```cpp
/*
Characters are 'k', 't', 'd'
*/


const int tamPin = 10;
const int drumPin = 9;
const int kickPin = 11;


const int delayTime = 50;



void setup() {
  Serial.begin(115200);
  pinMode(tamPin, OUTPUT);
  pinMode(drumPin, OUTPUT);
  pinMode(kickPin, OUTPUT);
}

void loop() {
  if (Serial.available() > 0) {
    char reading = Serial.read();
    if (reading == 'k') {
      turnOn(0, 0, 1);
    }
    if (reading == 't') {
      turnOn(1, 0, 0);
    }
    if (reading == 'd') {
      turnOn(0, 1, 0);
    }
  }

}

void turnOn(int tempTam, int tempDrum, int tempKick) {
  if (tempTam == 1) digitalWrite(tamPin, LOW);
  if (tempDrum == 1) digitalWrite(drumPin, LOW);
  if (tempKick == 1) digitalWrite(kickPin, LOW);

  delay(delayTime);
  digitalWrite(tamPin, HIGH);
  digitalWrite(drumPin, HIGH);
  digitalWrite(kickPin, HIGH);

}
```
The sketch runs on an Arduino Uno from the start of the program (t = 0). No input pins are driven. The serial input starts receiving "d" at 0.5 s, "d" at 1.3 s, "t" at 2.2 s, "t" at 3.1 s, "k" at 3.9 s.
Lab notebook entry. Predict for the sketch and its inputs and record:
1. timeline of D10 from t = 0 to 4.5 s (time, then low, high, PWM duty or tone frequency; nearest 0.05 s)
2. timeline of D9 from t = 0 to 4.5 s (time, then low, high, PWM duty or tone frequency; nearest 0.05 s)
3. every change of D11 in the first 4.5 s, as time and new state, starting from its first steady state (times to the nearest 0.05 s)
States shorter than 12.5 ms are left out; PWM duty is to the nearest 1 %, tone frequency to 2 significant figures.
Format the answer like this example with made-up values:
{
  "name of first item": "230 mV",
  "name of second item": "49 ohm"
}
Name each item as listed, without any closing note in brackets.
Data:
{
  "timeline of D10 from t = 0 to 4.5 s": "0 s low; 0.55 s high; 2.2 s low; 2.25 s high; 3.1 s low; 3.15 s high",
  "timeline of D9 from t = 0 to 4.5 s": "0 s low; 0.55 s high; 1.3 s low; 1.35 s high",
  "every change of D11 in the first 4.5 s, as time and new state, starting from its first steady state": "0 s low; 0.55 s high; 3.9 s low; 3.95 s high"
}
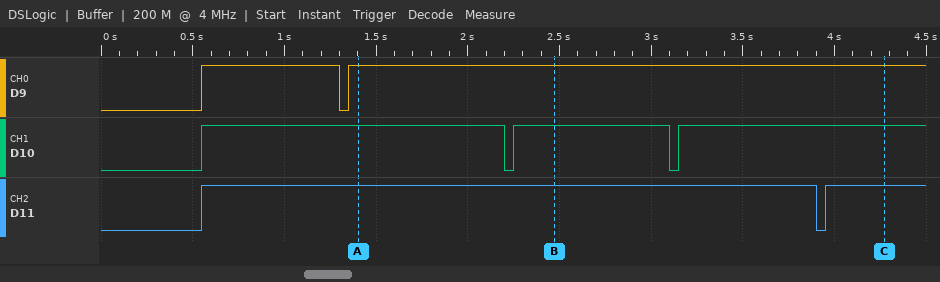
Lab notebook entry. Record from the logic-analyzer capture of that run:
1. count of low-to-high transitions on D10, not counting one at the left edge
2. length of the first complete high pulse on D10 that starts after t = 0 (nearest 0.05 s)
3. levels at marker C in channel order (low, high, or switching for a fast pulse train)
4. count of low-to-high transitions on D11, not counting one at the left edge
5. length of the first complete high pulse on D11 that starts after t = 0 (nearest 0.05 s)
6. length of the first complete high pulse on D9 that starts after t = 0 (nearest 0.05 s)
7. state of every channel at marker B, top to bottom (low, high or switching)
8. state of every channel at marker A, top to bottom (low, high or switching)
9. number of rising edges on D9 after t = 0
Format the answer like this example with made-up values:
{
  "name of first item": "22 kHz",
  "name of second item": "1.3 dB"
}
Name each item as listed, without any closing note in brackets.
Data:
{
  "count of low-to-high transitions on D10, not counting one at the left edge": "3",
  "length of the first complete high pulse on D10 that starts after t = 0": "1.65 s",
  "levels at marker C in channel order": "D9 high, D10 high, D11 high",
  "count of low-to-high transitions on D11, not counting one at the left edge": "2",
  "length of the first complete high pulse on D11 that starts after t = 0": "3.35 s",
  "length of the first complete high pulse on D9 that starts after t = 0": "0.75 s",
  "state of every channel at marker B, top to bottom": "D9 high, D10 high, D11 high",
  "state of every channel at marker A, top to bottom": "D9 high, D10 high, D11 high",
  "number of rising edges on D9 after t = 0": "2"
}
